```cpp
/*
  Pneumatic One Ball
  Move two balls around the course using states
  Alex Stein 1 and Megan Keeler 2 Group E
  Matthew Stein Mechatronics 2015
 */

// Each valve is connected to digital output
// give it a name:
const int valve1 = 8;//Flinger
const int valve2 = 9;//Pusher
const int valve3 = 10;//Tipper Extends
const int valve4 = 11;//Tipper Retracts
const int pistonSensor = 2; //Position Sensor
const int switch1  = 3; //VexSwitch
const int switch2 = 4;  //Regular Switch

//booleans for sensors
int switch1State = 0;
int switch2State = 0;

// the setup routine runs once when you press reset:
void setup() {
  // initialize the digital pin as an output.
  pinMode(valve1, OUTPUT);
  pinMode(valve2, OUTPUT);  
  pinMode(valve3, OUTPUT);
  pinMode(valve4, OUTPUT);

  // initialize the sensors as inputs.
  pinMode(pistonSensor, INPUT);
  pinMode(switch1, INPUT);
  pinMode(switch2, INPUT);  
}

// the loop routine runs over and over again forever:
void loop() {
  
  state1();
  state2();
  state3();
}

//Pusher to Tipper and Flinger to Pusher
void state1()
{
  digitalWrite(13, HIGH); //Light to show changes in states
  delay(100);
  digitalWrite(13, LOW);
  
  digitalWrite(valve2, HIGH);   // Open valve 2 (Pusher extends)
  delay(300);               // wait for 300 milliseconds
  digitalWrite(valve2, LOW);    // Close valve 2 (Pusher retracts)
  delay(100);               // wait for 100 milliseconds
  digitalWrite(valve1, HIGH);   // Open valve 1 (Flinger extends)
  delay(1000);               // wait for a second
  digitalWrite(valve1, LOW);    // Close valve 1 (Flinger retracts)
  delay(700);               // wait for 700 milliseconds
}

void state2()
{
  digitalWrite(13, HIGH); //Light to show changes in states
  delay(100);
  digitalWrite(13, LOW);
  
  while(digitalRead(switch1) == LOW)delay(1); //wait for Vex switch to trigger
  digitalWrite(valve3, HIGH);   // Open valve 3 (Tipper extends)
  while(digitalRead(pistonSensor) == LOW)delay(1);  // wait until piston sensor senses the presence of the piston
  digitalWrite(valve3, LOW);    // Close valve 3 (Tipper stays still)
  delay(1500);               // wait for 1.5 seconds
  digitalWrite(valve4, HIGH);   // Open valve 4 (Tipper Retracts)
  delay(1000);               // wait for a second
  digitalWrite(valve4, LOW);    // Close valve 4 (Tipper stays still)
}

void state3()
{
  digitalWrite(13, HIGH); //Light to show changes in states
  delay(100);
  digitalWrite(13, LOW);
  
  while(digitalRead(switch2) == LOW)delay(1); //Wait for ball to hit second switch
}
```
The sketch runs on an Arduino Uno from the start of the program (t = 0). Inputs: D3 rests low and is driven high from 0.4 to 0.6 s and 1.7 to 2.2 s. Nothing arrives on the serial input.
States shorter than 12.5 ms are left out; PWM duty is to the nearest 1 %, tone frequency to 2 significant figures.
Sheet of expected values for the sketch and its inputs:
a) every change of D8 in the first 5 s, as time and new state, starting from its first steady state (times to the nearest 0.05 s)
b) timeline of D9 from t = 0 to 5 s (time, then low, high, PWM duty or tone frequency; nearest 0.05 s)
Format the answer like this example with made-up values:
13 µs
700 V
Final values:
0 s low; 0.5 s high; 1.5 s low
0 s low; 0.1 s high; 0.4 s low
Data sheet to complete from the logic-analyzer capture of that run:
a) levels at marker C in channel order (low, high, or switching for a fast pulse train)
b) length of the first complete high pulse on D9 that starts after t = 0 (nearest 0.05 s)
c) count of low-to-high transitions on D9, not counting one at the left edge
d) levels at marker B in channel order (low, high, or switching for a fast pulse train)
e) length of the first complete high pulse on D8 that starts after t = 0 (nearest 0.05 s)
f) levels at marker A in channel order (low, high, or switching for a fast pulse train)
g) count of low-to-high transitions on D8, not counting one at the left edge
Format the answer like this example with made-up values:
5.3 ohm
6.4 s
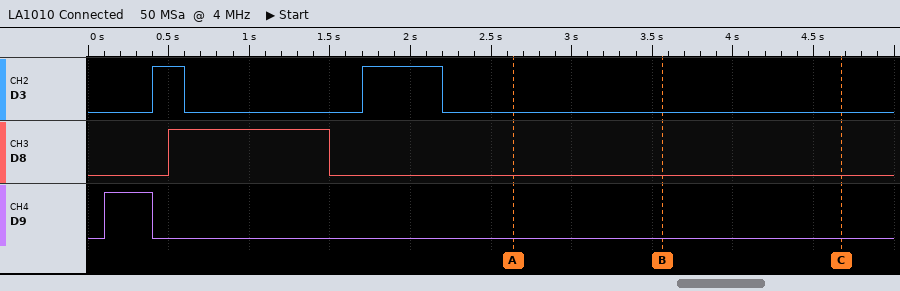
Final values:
D3 low, D8 low, D9 low
0.30 s
1
D3 low, D8 low, D9 low
1.00 s
D3 low, D8 low, D9 low
1
